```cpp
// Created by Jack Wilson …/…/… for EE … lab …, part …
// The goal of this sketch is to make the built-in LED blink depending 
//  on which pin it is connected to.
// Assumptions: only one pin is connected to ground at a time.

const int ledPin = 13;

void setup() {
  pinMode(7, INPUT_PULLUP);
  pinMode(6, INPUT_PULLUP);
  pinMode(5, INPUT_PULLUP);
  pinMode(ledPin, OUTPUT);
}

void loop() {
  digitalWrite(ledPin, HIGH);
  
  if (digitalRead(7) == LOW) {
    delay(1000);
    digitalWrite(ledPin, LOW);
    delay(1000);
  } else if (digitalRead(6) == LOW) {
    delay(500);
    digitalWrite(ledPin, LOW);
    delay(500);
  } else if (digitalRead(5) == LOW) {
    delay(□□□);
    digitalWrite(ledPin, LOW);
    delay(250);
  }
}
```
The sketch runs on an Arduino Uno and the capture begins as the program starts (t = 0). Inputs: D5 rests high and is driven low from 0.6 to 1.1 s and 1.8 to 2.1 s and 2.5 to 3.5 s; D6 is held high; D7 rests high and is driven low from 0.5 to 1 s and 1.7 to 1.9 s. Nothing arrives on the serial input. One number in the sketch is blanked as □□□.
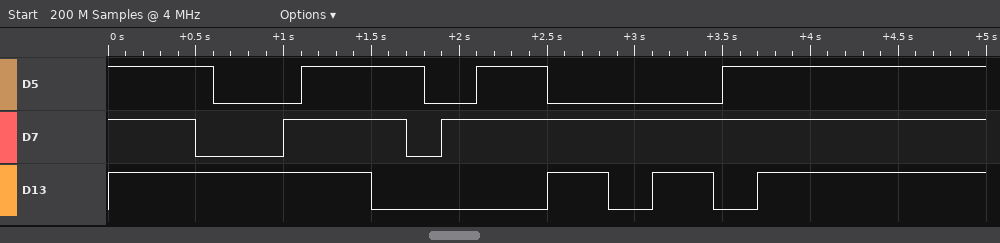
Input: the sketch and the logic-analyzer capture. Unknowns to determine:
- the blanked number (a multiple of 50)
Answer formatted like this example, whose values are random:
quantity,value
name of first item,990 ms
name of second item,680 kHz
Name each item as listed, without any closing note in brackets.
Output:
quantity,value
the blanked number,350
